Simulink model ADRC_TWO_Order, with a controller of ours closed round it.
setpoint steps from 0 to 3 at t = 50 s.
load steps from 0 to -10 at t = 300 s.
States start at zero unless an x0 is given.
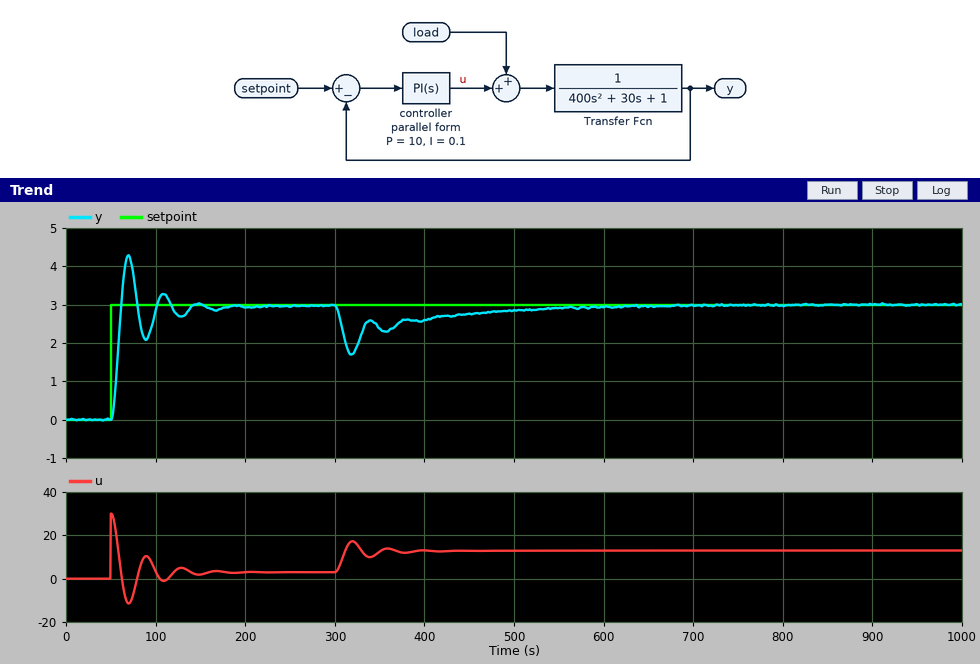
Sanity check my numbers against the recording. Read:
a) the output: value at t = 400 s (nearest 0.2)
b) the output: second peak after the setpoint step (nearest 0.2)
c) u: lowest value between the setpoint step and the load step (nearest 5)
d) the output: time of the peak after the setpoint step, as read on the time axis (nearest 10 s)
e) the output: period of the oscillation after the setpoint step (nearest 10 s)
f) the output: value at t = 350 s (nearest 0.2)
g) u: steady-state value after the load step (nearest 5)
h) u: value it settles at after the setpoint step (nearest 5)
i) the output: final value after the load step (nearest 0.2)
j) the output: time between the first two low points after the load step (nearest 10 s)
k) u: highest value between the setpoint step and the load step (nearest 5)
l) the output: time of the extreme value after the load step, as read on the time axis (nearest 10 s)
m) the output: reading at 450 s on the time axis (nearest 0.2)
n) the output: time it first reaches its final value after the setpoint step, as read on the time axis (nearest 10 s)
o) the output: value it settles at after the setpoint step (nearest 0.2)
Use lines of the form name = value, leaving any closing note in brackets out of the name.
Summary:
the output: value at t = 400 s = 2.6
the output: second peak after the setpoint step = 3.2
u: lowest value between the setpoint step and the load step = -10
the output: time of the peak after the setpoint step, as read on the time axis = 70 s
the output: period of the oscillation after the setpoint step = 40 s
the output: value at t = 350 s = 2.4
u: steady-state value after the load step = 15
u: value it settles at after the setpoint step = 5
the output: final value after the load step = 3.0
the output: time between the first two low points after the load step = 40 s
u: highest value between the setpoint step and the load step = 30
the output: time of the extreme value after the load step, as read on the time axis = 320 s
the output: reading at 450 s on the time axis = 2.8
the output: time it first reaches its final value after the setpoint step, as read on the time axis = 60 s
the output: value it settles at after the setpoint step = 3.0
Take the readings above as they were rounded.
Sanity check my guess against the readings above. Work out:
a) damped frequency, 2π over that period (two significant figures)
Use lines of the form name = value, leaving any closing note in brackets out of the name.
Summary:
damped frequency, 2π over that period = 0.16 rad/s
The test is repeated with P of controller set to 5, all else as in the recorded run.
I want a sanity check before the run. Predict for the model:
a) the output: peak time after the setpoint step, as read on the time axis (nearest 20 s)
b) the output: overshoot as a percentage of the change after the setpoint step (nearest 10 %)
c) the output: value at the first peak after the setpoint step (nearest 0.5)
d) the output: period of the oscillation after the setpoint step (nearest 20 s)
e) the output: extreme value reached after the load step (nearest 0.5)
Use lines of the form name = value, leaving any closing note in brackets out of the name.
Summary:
the output: peak time after the setpoint step, as read on the time axis = 80 s
the output: overshoot as a percentage of the change after the setpoint step = 30 %
the output: value at the first peak after the setpoint step = 4.0
the output: period of the oscillation after the setpoint step = 60 s
the output: extreme value reached after the load step = 1.0
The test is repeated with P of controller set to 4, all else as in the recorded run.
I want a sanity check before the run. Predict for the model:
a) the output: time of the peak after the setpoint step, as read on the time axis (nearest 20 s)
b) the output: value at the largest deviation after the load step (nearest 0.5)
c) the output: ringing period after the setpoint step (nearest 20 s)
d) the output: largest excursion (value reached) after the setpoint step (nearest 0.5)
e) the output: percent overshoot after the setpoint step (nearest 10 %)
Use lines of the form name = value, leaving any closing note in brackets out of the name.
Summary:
the output: time of the peak after the setpoint step, as read on the time axis = 80 s
the output: value at the largest deviation after the load step = 0.5
the output: ringing period after the setpoint step = 60 s
the output: largest excursion (value reached) after the setpoint step = 4.0
the output: percent overshoot after the setpoint step = 30 %
